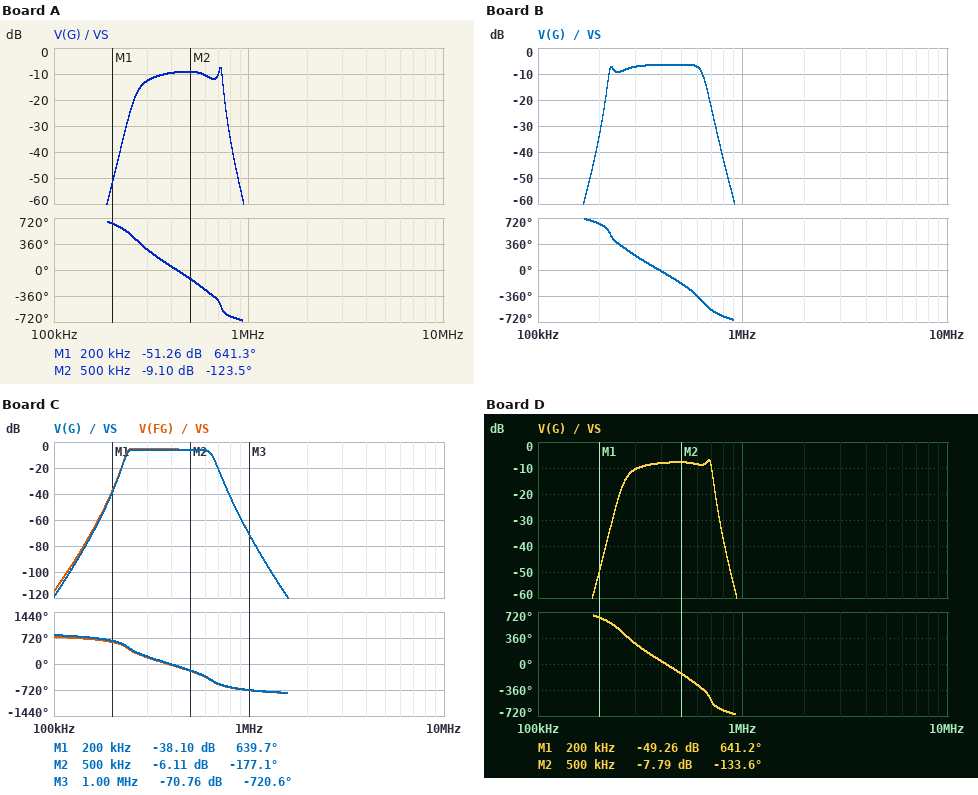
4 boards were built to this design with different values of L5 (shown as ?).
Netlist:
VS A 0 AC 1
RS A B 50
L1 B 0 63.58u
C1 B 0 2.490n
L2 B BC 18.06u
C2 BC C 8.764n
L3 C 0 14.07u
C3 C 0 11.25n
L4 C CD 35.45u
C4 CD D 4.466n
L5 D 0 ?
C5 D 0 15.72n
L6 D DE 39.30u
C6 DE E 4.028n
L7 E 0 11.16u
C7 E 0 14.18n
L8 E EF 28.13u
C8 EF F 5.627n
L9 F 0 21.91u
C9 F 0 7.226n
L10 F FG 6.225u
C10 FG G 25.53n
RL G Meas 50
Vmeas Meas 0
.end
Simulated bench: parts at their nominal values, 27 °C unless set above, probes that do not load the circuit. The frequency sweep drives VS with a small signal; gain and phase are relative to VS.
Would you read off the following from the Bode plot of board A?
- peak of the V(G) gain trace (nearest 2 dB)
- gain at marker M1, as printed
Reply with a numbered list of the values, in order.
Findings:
1. -8 dB
2. -51.26 dB
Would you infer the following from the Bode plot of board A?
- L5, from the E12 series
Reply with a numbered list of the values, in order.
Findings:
1. 4.7 µH
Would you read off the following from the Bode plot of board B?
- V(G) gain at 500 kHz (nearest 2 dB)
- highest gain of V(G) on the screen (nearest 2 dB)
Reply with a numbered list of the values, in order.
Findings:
1. -6 dB
2. -6 dB
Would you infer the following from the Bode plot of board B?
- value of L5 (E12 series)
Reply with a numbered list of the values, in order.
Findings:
1. 15 µH
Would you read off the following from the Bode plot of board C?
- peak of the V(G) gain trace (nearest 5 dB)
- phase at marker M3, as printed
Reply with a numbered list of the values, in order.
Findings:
1. -5 dB
2. -720.6 deg
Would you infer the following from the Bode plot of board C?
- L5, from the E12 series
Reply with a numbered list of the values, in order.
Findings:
1. 12 µH
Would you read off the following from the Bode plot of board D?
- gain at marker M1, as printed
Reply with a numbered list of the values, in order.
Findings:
1. -49.26 dB
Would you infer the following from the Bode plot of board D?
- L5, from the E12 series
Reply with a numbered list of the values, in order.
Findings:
1. 5.6 µH
